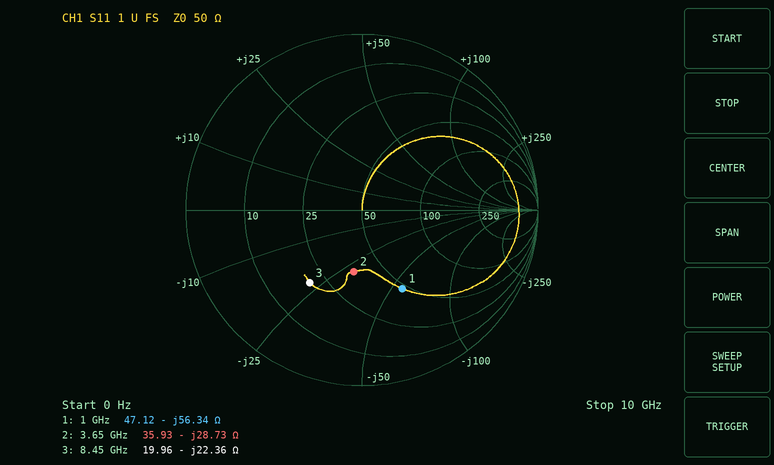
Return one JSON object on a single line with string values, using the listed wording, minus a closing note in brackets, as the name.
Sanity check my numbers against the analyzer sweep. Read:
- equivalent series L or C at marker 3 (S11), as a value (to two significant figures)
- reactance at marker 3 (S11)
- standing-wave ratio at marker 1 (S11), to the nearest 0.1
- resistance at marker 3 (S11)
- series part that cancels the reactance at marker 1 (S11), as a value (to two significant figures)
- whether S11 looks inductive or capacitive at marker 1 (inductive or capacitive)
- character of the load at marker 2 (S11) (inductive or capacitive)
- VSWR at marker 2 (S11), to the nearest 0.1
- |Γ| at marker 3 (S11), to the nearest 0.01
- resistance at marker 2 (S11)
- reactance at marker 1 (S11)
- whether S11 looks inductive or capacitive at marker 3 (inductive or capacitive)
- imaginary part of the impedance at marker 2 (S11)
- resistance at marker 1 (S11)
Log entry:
{"equivalent series L or C at marker 3 (S11), as a value": "840 fF", "reactance at marker 3": "-22.36 Ω", "standing-wave ratio at marker 1 (S11), to the nearest 0.1": "3.0", "resistance at marker 3": "19.96 Ω", "series part that cancels the reactance at marker 1 (S11), as a value": "9.0 nH", "whether S11 looks inductive or capacitive at marker 1": "capacitive", "character of the load at marker 2 (S11)": "capacitive", "VSWR at marker 2 (S11), to the nearest 0.1": "2.1", "|Γ| at marker 3 (S11), to the nearest 0.01": "0.51", "resistance at marker 2": "35.93 Ω", "reactance at marker 1": "-56.34 Ω", "whether S11 looks inductive or capacitive at marker 3": "capacitive", "imaginary part of the impedance at marker 2": "-28.73 Ω", "resistance at marker 1": "47.12 Ω"}
